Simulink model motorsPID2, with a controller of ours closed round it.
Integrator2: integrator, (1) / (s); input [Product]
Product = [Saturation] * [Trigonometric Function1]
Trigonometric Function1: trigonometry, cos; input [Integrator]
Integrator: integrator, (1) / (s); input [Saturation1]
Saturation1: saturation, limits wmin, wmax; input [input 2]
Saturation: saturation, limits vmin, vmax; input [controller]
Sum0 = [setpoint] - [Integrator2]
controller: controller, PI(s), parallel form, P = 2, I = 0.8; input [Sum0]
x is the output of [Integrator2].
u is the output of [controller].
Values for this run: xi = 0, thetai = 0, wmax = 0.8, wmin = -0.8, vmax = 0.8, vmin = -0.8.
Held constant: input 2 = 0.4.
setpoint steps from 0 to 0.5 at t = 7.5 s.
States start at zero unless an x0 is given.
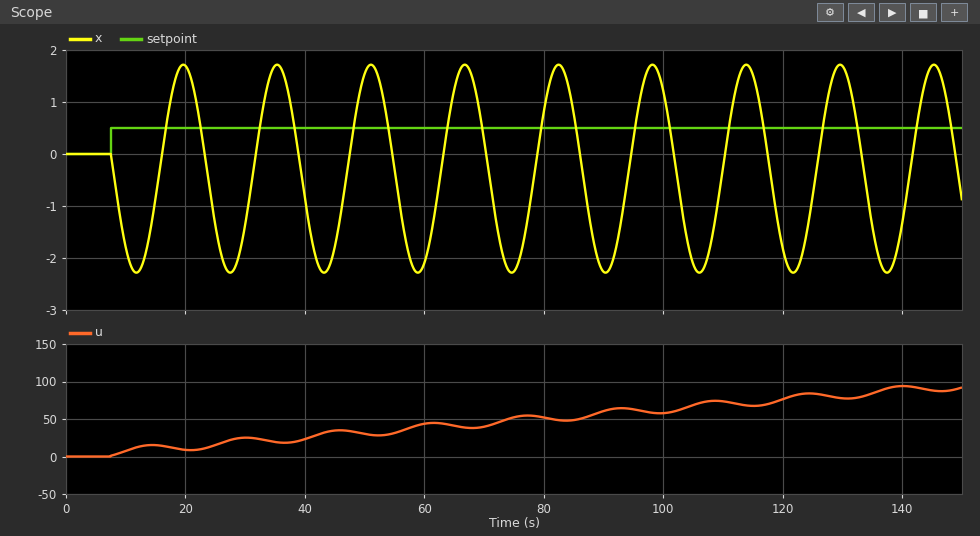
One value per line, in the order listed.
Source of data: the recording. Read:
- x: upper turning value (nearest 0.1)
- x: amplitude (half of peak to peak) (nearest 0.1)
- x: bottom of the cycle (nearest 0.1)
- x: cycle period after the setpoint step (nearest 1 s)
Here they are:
1.7
2.0
-2.3
16 s
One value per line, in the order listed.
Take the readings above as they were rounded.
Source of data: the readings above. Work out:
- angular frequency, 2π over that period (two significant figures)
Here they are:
0.39 rad/s
